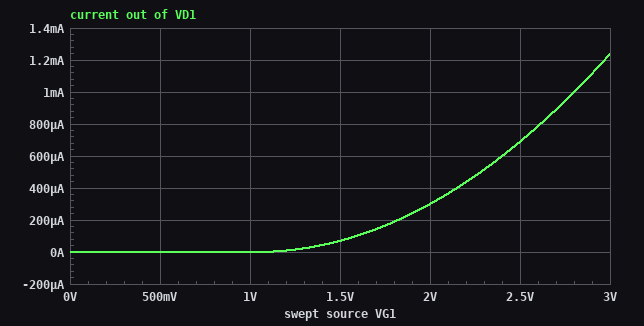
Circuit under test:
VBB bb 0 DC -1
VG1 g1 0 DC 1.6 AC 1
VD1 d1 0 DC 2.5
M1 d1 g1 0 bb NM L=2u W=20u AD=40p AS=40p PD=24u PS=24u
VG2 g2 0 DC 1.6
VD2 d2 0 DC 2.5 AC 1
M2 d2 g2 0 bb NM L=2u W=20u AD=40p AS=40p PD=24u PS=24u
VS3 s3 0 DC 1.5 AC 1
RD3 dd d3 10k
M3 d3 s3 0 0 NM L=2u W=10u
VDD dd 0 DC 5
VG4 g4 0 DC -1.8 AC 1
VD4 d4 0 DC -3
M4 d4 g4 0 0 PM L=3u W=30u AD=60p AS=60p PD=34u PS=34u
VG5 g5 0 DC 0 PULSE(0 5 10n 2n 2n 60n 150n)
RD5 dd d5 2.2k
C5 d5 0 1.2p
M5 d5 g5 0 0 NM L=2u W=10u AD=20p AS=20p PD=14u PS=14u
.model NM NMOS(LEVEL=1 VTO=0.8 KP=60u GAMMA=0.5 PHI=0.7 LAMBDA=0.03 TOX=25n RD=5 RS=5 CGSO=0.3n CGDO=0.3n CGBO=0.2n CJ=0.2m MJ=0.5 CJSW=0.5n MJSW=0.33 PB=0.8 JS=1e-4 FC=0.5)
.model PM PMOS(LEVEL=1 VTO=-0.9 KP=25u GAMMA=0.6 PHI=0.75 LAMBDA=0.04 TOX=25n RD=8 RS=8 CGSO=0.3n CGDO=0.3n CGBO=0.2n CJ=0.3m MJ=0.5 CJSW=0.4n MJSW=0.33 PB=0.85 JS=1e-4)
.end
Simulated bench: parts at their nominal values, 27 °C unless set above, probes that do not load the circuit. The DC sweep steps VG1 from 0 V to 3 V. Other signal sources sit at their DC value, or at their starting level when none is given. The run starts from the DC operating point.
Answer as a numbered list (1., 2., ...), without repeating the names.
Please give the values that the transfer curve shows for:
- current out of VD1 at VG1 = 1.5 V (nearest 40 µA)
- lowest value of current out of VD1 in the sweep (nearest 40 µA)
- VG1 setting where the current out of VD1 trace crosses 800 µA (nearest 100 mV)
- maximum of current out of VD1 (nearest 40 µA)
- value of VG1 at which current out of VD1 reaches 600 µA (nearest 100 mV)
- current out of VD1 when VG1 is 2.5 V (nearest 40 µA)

1. 80 µA
2. 0 A
3. 2.6 V
4. 1.24 mA
5. 2.4 V
6. 680 µA
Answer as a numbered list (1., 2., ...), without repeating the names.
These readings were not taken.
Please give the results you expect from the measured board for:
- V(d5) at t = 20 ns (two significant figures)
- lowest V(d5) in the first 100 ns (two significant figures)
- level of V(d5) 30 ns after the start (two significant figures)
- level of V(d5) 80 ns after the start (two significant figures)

1. 1.5 V
2. 1.5 V
3. 1.5 V
4. 4.8 V
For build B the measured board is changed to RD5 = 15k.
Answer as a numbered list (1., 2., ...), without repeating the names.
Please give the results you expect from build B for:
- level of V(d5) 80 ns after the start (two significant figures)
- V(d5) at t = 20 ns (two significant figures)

1. 1.8 V
2. 260 mV
